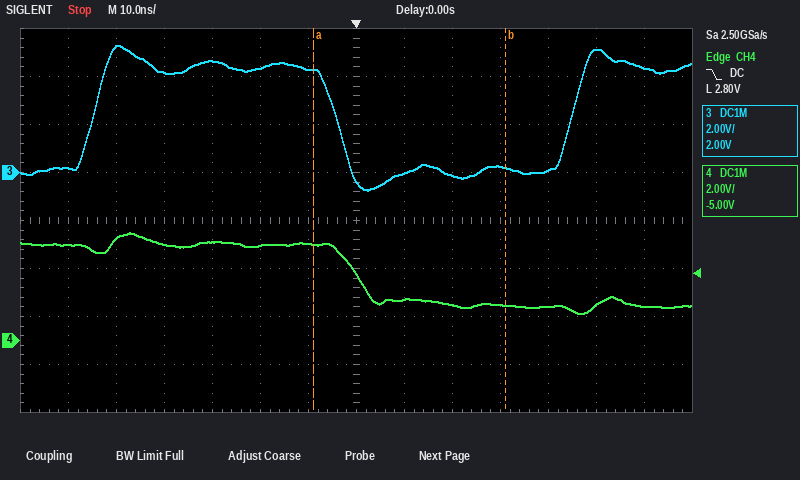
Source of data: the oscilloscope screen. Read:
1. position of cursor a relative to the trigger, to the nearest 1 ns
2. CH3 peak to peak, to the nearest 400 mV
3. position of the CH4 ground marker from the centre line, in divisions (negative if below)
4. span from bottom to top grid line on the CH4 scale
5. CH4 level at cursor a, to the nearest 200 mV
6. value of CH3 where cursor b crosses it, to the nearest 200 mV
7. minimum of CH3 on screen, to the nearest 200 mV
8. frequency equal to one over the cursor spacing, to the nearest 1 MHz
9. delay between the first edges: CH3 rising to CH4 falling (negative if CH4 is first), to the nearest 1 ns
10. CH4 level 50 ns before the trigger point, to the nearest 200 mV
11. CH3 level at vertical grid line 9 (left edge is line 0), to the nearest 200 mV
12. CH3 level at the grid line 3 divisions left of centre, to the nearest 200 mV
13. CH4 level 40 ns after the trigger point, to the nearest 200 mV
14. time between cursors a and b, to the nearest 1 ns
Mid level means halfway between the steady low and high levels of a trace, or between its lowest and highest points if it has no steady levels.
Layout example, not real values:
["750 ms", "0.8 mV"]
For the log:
["-9 ns", "6.0 V", "-2.5 div", "16 V", "4.0 V", "200 mV", "-800 mV", "25 MHz", "+55 ns", "4.2 V", "-200 mV", "4.6 V", "1.4 V", "40 ns"]
